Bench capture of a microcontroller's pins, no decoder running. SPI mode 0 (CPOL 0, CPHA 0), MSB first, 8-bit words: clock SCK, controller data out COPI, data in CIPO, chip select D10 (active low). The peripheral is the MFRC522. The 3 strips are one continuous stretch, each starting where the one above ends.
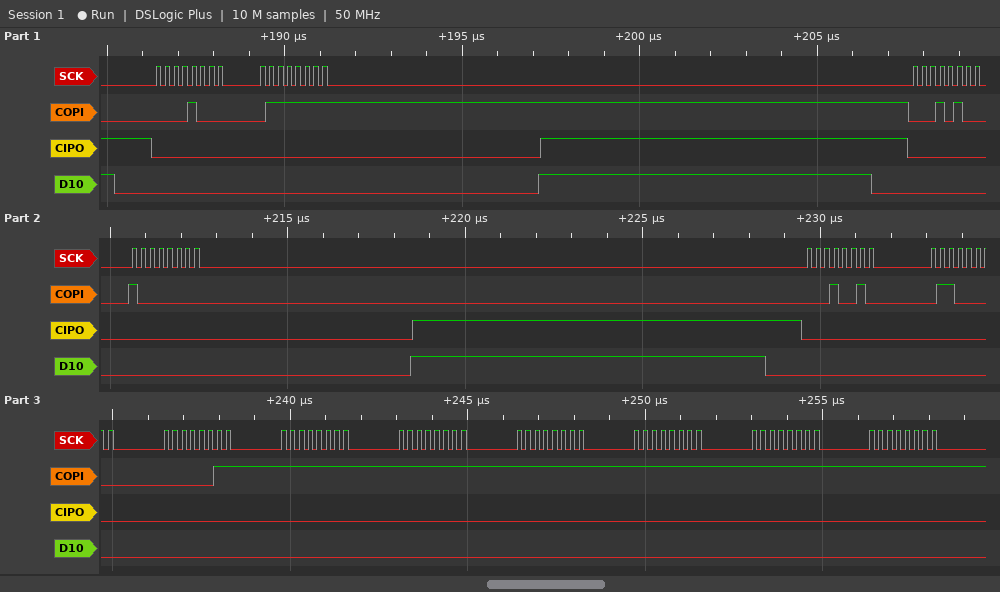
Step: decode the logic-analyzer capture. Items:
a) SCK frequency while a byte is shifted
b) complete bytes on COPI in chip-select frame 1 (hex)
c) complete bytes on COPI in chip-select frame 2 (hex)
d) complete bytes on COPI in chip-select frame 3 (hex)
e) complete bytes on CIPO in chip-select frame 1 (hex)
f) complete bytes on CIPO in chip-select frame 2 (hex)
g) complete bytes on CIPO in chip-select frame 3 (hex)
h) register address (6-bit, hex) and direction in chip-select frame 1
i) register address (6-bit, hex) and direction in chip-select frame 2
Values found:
4 MHz
0x08 0x7F
0x14 0x80
0x12 0x60 0x03 0xFF 0xFF 0xFF 0xFF 0xFF 0xFF
0x00 0x00
0x00 0x00
0x00 0x00 0x00 0x00 0x00 0x00 0x00 0x00 0x00
0x04 write
0x0A write
